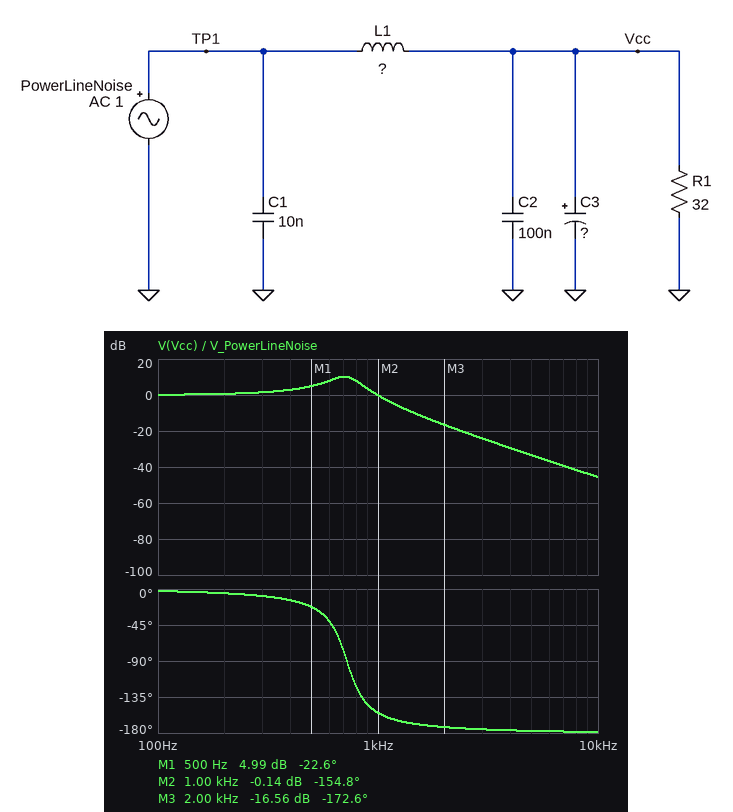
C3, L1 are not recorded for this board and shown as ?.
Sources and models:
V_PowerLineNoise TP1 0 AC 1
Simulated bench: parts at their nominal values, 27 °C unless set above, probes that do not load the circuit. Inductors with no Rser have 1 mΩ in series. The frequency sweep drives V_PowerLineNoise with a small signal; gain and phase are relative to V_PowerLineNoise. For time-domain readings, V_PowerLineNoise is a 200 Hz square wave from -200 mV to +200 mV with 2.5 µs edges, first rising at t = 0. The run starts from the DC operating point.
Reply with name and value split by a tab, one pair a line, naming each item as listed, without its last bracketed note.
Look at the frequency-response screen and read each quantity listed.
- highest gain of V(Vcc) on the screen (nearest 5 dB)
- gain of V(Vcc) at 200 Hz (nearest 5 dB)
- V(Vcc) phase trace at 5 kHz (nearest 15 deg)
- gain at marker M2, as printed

highest gain of V(Vcc) on the screen	10 dB
gain of V(Vcc) at 200 Hz	0 dB
V(Vcc) phase trace at 5 kHz	-180 deg
gain at marker M2, as printed	-0.14 dB
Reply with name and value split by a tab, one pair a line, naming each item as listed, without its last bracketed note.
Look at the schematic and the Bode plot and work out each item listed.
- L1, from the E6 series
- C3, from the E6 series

L1, from the E6 series	2.2 mH
C3, from the E6 series	22 µF
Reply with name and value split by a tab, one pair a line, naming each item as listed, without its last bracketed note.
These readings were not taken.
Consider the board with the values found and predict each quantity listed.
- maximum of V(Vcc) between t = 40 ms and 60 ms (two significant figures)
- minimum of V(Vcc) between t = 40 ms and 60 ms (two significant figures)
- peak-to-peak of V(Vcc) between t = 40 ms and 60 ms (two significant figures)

maximum of V(Vcc) between t = 40 ms and 60 ms	440 mV
minimum of V(Vcc) between t = 40 ms and 60 ms	-440 mV
peak-to-peak of V(Vcc) between t = 40 ms and 60 ms	880 mV
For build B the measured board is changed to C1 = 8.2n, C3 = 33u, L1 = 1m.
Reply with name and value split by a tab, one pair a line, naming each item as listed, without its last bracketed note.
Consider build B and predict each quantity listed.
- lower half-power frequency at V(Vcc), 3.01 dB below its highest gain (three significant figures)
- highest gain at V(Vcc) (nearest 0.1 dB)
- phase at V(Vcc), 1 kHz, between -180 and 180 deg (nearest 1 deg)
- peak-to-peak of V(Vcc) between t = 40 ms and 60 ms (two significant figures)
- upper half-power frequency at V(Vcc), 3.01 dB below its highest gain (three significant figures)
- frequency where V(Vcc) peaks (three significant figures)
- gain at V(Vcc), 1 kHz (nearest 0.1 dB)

lower half-power frequency at V(Vcc), 3.01 dB below its highest gain	789 Hz
highest gain at V(Vcc)	15.3 dB
phase at V(Vcc), 1 kHz, between -180 and 180 deg	-147 deg
peak-to-peak of V(Vcc) between t = 40 ms and 60 ms	910 mV
upper half-power frequency at V(Vcc), 3.01 dB below its highest gain	941 Hz
frequency where V(Vcc) peaks	868 Hz
gain at V(Vcc), 1 kHz	8.8 dB
